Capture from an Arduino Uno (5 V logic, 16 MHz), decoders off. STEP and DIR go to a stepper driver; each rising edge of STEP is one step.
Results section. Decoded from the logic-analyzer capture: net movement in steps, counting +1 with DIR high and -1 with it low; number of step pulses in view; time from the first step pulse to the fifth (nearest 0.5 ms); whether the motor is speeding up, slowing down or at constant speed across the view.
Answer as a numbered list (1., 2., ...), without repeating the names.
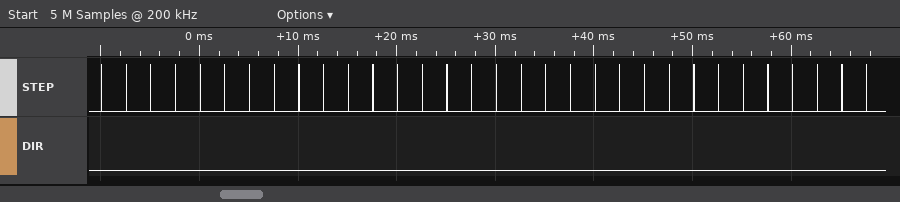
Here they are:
1. -32
2. 32
3. 10.0 ms
4. constant speed
